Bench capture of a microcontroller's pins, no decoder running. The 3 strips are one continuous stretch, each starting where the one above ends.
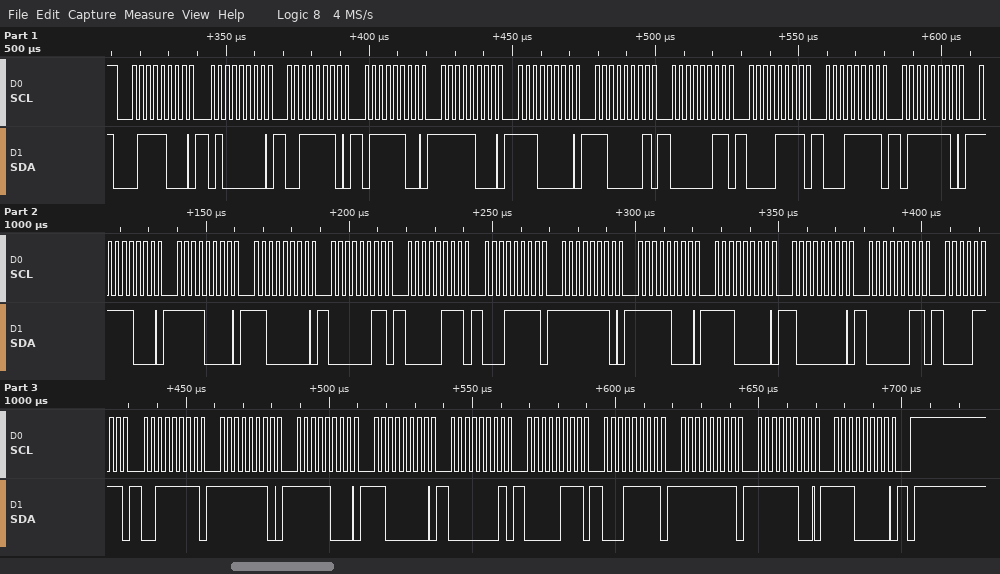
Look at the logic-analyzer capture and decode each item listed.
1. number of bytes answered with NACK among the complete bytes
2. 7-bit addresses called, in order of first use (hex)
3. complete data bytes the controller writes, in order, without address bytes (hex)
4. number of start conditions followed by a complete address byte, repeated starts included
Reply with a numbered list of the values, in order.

1. 0
2. 0x3C
3. 40 3E 7C F8 E0 C1 03 0F 1F 7E F8 F0 C0 03 07 1F FE F8 E0 80 03 0F 3F FE F8 C0 01 07 1F FF FC E0
4. 1
